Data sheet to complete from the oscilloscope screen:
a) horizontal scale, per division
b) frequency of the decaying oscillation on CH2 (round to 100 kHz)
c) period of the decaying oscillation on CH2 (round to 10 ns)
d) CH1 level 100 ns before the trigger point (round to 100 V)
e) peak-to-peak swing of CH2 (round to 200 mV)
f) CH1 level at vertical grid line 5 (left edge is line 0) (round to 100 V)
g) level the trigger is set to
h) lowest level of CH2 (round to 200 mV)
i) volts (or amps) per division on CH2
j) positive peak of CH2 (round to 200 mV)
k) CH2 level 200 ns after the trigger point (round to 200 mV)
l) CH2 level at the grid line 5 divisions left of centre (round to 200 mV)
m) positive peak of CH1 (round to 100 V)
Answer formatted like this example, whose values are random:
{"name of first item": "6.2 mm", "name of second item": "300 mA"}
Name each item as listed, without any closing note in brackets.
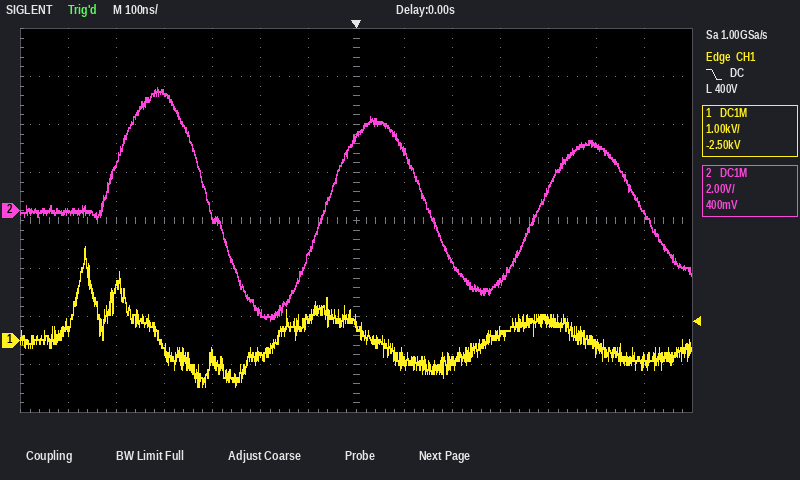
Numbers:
{"horizontal scale, per division": "100 ns", "frequency of the decaying oscillation on CH2": "2.2 MHz", "period of the decaying oscillation on CH2": "450 ns", "CH1 level 100 ns before the trigger point": "500 V", "peak-to-peak swing of CH2": "9.8 V", "CH1 level at vertical grid line 5 (left edge is line 0)": "-300 V", "level the trigger is set to": "400 V", "lowest level of CH2": "-4.6 V", "volts (or amps) per division on CH2": "2 V", "positive peak of CH2": "5.2 V", "CH2 level 200 ns after the trigger point": "-2.2 V", "CH2 level at the grid line 5 divisions left of centre": "2.0 V", "positive peak of CH1": "2.0 kV"}
